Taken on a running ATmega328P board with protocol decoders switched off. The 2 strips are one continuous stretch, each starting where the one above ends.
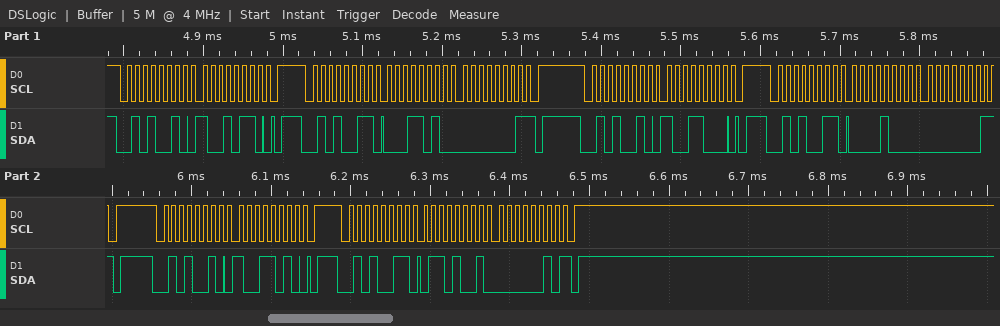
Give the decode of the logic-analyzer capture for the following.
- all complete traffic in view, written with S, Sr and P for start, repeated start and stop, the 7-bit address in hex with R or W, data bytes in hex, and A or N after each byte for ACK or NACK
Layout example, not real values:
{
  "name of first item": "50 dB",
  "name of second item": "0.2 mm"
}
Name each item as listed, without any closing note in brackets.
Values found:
{
  "all complete traffic in view, written with S, Sr and P for start, repeated start and stop, the 7-bit address in hex with R or W, data bytes in hex, and A or N after each byte for ACK or NACK": "S 29W A 96 A P S 29R A 1A A 01 N P S 29W A 98 A P S 29R A 08 A 01 N P S 29W A 9A A P S 29R A 69 A 02 N P"
}
